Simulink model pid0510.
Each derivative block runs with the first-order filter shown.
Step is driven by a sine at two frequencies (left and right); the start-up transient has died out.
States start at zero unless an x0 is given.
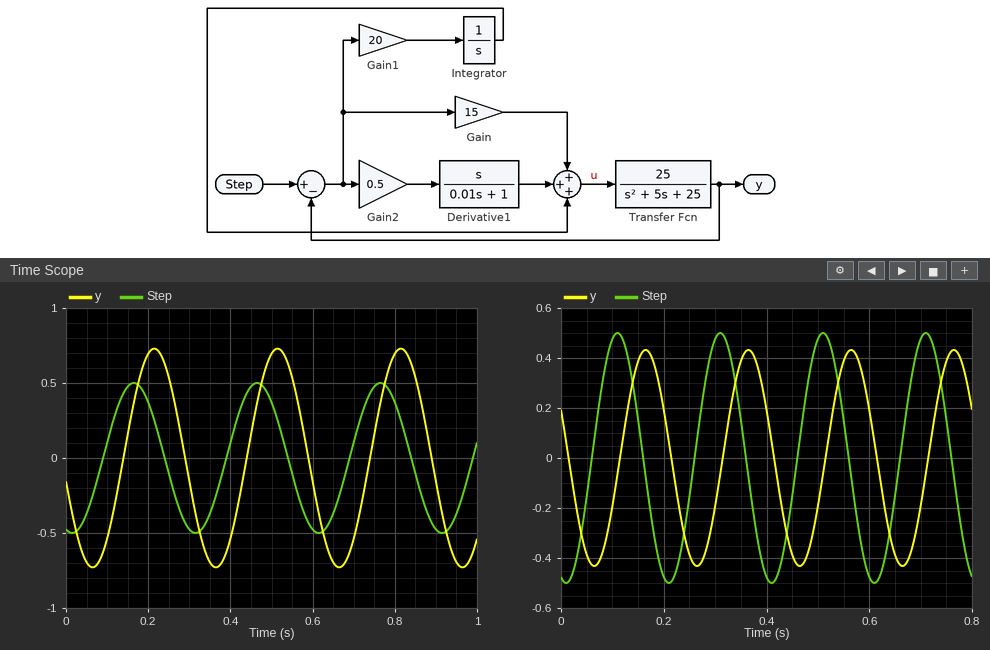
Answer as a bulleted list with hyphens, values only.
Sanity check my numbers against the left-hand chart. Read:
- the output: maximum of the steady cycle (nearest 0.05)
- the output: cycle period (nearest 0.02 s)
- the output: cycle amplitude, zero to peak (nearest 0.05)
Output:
- 0.75
- 0.30 s
- 0.75
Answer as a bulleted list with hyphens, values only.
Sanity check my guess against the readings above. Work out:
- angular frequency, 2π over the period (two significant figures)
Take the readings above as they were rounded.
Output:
- 21 rad/s
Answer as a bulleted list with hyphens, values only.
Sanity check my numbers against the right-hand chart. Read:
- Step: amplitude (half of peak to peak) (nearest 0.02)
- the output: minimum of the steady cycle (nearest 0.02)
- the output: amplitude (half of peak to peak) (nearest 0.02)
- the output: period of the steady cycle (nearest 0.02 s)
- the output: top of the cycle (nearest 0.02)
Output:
- 0.50
- -0.44
- 0.44
- 0.20 s
- 0.44
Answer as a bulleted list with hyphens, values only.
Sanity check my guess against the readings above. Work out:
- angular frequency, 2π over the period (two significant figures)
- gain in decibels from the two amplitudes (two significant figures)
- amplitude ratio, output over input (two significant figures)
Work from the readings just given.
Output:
- 31 rad/s
- -1.1 dB
- 0.88
